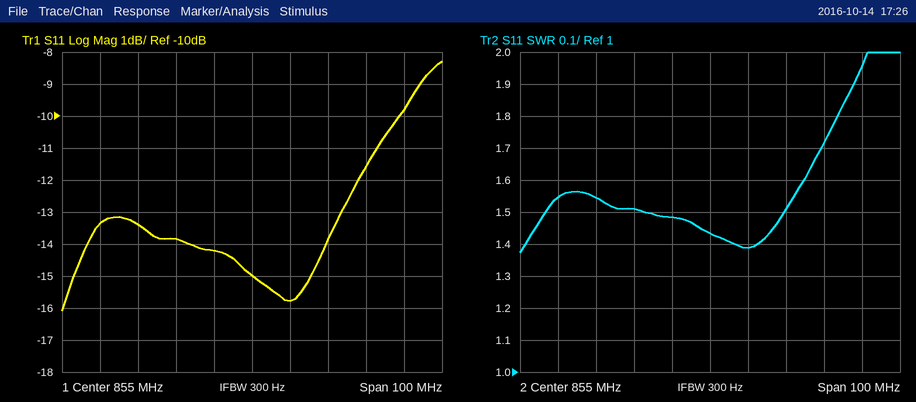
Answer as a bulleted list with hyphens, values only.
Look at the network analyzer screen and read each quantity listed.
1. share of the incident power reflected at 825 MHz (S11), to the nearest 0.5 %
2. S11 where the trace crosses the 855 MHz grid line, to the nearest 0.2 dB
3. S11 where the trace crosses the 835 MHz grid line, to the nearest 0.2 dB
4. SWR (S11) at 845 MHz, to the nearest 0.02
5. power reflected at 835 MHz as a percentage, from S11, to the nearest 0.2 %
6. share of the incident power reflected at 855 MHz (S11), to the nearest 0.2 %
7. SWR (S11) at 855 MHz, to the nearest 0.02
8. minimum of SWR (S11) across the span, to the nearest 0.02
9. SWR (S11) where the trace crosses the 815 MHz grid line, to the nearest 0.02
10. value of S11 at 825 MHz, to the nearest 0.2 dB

- 4.5 %
- -15.0 dB
- -13.8 dB
- 1.48
- 4.2 %
- 3.2 %
- 1.44
- 1.38
- 1.54
- -13.4 dB
